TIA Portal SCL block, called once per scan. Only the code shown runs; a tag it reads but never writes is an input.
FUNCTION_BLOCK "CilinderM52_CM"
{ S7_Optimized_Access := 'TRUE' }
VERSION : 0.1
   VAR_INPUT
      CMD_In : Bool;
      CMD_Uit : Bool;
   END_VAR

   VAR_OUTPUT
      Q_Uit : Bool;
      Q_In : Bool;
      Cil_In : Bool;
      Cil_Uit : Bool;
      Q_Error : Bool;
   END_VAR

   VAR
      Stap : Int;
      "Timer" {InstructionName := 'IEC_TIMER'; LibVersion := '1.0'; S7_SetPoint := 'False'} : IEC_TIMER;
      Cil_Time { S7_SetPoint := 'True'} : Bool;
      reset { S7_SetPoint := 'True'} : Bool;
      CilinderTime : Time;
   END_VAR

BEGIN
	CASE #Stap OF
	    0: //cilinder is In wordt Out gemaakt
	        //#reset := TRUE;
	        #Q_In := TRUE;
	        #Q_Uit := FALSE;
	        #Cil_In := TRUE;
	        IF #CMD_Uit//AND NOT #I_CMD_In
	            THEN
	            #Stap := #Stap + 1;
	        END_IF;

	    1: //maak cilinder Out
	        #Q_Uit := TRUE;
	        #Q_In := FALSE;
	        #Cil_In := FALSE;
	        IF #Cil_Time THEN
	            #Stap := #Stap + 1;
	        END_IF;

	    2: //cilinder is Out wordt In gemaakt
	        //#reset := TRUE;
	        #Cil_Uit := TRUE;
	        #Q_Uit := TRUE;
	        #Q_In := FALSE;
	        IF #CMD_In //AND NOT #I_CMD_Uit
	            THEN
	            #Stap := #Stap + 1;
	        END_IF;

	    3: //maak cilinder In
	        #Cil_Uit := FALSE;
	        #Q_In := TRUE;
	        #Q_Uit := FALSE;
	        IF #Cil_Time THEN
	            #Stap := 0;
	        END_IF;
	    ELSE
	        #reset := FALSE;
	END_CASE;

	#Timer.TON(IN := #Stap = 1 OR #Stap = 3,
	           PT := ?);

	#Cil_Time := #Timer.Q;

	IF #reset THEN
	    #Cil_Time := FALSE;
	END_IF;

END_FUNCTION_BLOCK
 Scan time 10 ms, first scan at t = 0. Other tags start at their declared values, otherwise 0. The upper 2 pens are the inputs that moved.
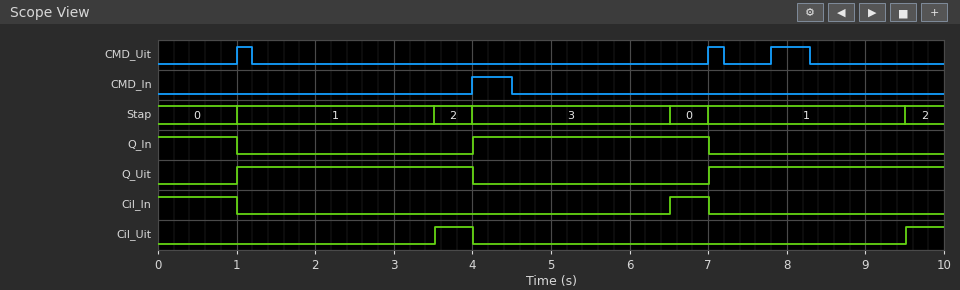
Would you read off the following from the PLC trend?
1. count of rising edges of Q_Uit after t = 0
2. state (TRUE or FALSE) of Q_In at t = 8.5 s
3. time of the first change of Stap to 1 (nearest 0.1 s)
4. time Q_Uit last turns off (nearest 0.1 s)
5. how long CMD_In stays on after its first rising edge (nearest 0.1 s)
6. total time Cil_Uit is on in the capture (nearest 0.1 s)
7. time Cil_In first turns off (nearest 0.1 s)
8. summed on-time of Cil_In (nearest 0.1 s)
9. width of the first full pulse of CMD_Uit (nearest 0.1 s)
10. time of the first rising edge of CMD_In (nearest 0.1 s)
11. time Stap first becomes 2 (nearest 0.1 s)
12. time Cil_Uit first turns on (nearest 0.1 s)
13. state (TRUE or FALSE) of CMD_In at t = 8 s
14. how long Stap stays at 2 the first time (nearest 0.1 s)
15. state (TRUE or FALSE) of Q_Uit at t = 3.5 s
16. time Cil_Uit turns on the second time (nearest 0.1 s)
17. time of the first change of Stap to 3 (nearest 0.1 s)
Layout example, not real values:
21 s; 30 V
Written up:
2; FALSE; 1.0 s; 4.0 s; 0.5 s; 1.0 s; 1.0 s; 1.5 s; 0.2 s; 4.0 s; 3.5 s; 3.5 s; FALSE; 0.5 s; TRUE; 9.5 s; 4.0 s
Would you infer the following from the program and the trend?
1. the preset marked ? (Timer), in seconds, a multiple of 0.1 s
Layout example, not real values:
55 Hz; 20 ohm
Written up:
2.5 s
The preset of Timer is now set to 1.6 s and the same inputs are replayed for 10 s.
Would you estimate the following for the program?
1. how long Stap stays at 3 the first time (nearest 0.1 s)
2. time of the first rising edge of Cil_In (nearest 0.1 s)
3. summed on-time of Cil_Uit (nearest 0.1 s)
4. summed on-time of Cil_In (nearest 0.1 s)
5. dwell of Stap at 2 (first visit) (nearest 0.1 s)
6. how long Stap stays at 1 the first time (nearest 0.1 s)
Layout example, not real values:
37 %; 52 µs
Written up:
1.6 s; 5.6 s; 2.8 s; 2.4 s; 1.4 s; 1.6 s
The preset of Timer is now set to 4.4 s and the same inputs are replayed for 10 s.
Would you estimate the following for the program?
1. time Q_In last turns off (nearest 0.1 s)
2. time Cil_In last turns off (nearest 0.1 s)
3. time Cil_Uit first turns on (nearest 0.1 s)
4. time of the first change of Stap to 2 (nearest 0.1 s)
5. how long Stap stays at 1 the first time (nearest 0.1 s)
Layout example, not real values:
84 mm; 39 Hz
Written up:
1.0 s; 1.0 s; 5.4 s; 5.4 s; 4.4 s
